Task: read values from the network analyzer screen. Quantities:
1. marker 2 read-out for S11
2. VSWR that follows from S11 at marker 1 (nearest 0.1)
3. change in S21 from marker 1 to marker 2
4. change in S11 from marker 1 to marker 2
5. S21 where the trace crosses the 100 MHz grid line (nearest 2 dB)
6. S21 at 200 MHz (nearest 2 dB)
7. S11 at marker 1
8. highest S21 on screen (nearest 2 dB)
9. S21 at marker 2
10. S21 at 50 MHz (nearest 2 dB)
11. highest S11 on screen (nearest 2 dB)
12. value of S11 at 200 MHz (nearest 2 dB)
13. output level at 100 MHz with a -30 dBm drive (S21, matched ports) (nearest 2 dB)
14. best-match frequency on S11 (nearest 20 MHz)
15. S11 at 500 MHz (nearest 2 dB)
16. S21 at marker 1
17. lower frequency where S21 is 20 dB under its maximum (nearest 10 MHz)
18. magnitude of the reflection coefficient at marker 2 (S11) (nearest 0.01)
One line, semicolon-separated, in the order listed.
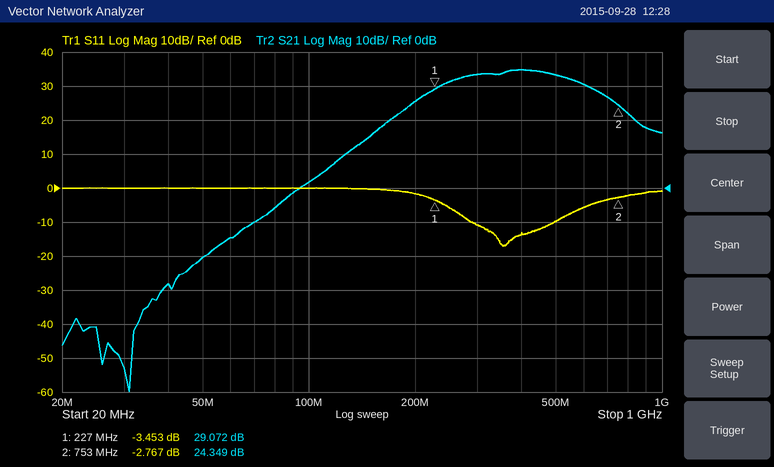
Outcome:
-2.767 dB; 5.1; -4.723 dB; 0.686 dB; 2 dB; 26 dB; -3.453 dB; 34 dB; 24.349 dB; -20 dB; 0 dB; -2 dB; -28 dBm; 360 MHz; -10 dB; 29.072 dB; 150 MHz; 0.73
